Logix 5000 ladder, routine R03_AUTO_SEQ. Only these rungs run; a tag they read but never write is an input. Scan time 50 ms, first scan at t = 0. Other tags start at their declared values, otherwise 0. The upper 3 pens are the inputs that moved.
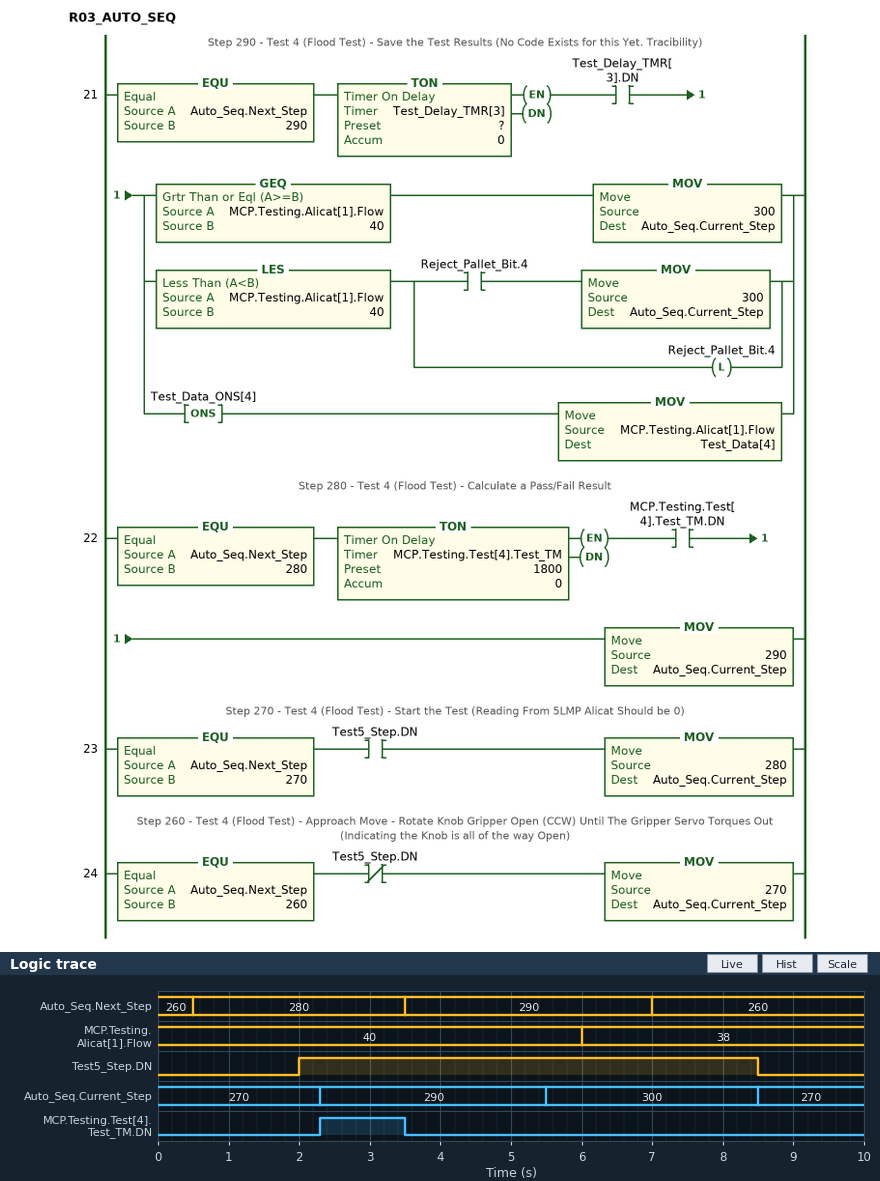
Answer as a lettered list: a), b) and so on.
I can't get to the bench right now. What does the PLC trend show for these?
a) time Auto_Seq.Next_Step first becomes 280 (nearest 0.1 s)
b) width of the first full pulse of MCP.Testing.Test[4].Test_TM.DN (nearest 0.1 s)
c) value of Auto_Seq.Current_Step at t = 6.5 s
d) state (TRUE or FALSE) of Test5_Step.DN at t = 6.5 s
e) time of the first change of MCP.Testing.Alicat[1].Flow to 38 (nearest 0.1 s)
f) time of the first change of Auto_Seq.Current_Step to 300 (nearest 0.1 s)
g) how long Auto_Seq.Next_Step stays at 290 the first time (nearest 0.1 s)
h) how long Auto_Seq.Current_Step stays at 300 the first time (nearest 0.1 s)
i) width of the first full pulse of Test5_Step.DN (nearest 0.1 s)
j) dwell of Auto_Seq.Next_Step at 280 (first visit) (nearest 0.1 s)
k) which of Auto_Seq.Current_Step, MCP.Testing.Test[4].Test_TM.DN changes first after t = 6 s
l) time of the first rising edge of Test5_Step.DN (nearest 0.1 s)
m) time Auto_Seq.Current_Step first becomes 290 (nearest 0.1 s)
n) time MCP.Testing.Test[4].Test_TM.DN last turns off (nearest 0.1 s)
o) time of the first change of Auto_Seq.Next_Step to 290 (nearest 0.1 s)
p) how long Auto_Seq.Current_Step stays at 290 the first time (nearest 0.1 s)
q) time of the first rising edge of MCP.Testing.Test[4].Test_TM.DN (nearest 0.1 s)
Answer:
a) 0.5 s
b) 1.2 s
c) 300
d) TRUE
e) 6.0 s
f) 5.5 s
g) 3.5 s
h) 3.0 s
i) 6.5 s
j) 3.0 s
k) Auto_Seq.Current_Step
l) 2.0 s
m) 2.3 s
n) 3.5 s
o) 3.5 s
p) 3.2 s
q) 2.3 s
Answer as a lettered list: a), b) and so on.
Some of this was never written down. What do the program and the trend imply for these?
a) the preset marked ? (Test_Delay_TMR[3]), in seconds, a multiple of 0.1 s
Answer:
a) 2.0 s
